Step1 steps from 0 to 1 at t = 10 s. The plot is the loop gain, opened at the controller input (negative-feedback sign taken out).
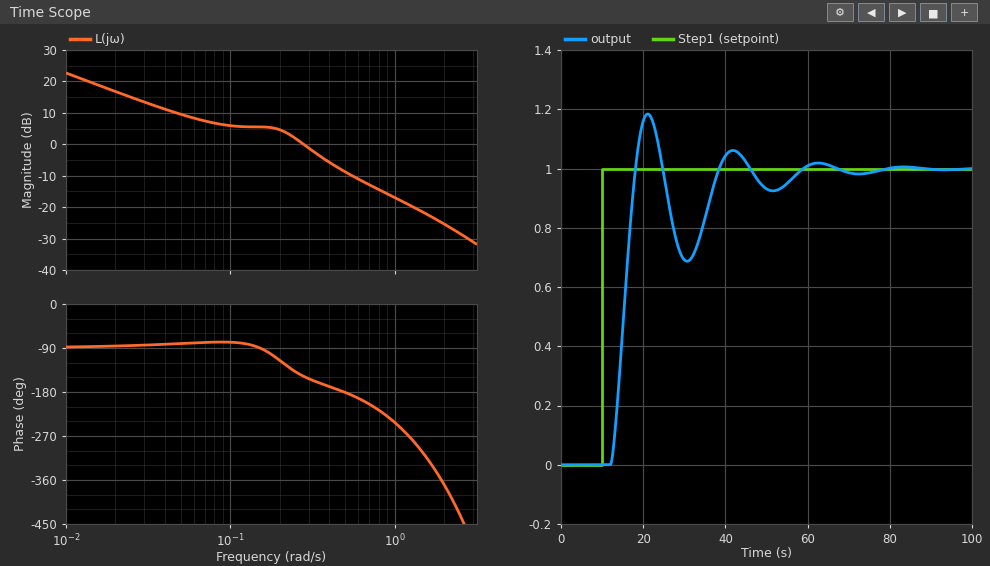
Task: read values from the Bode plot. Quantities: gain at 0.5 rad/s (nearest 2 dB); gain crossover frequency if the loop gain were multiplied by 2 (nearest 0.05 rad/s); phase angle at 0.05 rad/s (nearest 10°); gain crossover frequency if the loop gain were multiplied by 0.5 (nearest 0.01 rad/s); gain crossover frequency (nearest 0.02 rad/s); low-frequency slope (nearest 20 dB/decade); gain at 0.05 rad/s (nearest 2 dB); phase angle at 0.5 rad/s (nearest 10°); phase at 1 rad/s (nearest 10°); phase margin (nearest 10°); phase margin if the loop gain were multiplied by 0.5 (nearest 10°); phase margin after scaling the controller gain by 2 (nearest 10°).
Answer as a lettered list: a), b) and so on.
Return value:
a) -8 dB
b) 0.40 rad/s
c) -80°
d) 0.10 rad/s
e) 0.28 rad/s
f) -20 dB/decade
g) 10 dB
h) -180°
i) -240°
j) 30°
k) 100°
l) 10°
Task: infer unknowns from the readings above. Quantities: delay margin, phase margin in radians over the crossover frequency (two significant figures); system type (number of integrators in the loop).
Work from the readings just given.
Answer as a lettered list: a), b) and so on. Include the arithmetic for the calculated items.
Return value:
a) 30 × π / 180 / 0.28 = 1.9 s
b) 1
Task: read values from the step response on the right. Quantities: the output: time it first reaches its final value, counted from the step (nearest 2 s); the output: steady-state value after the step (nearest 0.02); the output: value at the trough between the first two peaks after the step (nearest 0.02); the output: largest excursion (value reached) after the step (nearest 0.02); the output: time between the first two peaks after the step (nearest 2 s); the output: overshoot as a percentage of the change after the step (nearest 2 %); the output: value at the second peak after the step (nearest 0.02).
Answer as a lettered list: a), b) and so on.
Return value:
a) 8 s
b) 1.00
c) 0.68
d) 1.18
e) 20 s
f) 18 %
g) 1.06
